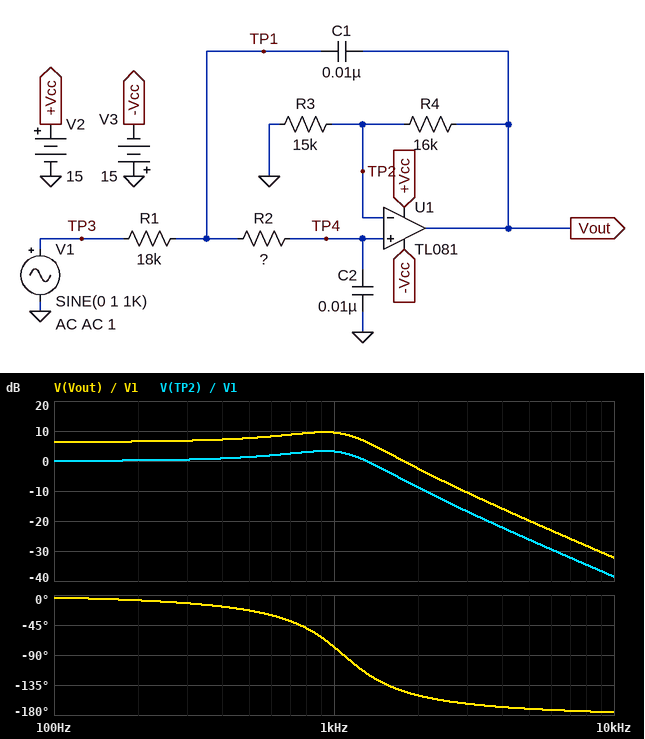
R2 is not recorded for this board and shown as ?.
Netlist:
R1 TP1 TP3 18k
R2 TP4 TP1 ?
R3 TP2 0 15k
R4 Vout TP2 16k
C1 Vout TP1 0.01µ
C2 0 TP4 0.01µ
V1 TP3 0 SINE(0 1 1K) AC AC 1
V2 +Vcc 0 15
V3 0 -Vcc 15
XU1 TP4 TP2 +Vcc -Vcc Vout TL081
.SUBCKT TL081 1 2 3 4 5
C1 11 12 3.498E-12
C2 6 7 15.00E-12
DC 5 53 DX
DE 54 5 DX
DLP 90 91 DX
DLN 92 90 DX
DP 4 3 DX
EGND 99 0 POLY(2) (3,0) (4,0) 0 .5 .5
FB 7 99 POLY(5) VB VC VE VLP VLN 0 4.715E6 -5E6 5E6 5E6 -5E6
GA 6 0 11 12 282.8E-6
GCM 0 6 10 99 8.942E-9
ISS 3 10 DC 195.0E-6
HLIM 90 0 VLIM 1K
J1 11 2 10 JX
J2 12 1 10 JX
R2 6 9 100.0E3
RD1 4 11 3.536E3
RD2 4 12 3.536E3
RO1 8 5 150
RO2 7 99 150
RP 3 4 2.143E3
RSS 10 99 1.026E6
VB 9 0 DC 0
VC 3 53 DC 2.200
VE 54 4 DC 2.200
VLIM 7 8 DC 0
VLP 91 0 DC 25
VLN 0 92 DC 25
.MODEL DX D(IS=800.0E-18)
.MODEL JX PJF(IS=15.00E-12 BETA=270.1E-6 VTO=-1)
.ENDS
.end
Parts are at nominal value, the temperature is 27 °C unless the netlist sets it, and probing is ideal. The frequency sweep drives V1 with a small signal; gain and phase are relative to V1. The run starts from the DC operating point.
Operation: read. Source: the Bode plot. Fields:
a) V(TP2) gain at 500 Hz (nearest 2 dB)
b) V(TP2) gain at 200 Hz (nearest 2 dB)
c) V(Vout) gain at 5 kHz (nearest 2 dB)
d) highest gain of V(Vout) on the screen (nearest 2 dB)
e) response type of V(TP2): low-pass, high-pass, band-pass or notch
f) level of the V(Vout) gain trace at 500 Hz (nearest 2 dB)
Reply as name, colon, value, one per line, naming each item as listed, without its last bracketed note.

V(TP2) gain at 500 Hz: 2 dB
V(TP2) gain at 200 Hz: 0 dB
V(Vout) gain at 5 kHz: -20 dB
highest gain of V(Vout) on the screen: 10 dB
response type of V(TP2): low-pass, high-pass, band-pass or notch: low-pass
level of the V(Vout) gain trace at 500 Hz: 8 dB
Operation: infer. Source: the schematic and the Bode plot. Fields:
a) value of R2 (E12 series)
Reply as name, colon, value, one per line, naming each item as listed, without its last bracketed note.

value of R2: 12 kΩ
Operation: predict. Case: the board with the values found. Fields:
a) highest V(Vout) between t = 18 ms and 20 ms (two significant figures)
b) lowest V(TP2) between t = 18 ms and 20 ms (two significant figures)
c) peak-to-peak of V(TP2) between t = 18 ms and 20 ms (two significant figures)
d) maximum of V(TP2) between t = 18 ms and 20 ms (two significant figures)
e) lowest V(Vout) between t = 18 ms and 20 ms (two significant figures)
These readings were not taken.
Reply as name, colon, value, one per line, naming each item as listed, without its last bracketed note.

highest V(Vout) between t = 18 ms and 20 ms: 3.0 V
lowest V(TP2) between t = 18 ms and 20 ms: -1.4 V
peak-to-peak of V(TP2) between t = 18 ms and 20 ms: 2.9 V
maximum of V(TP2) between t = 18 ms and 20 ms: 1.4 V
lowest V(Vout) between t = 18 ms and 20 ms: -3.0 V
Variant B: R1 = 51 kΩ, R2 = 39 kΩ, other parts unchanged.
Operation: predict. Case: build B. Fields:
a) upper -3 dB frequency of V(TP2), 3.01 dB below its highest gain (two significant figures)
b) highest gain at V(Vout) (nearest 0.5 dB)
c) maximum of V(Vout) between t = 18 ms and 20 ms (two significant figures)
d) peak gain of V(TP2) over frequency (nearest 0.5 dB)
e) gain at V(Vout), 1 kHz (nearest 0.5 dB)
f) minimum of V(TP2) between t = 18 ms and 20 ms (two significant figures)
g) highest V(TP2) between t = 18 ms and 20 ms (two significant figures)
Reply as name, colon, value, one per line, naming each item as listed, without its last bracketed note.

upper -3 dB frequency of V(TP2), 3.01 dB below its highest gain: 420 Hz
highest gain at V(Vout): 9.0 dB
maximum of V(Vout) between t = 18 ms and 20 ms: 290 mV
peak gain of V(TP2) over frequency: 2.5 dB
gain at V(Vout), 1 kHz: -11.0 dB
minimum of V(TP2) between t = 18 ms and 20 ms: -140 mV
highest V(TP2) between t = 18 ms and 20 ms: 140 mV
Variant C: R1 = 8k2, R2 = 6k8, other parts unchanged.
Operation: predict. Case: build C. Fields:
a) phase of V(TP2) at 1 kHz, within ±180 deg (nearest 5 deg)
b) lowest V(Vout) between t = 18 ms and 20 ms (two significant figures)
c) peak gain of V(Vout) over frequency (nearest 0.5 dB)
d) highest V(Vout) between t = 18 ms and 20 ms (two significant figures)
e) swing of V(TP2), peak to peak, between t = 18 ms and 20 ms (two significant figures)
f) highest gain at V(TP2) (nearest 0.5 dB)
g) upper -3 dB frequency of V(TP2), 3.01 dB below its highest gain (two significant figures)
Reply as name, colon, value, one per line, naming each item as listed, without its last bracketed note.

phase of V(TP2) at 1 kHz, within ±180 deg: -25 deg
lowest V(Vout) between t = 18 ms and 20 ms: -2.4 V
peak gain of V(Vout) over frequency: 8.5 dB
highest V(Vout) between t = 18 ms and 20 ms: 2.4 V
swing of V(TP2), peak to peak, between t = 18 ms and 20 ms: 2.3 V
highest gain at V(TP2): 2.5 dB
upper -3 dB frequency of V(TP2), 3.01 dB below its highest gain: 2.5 kHz
